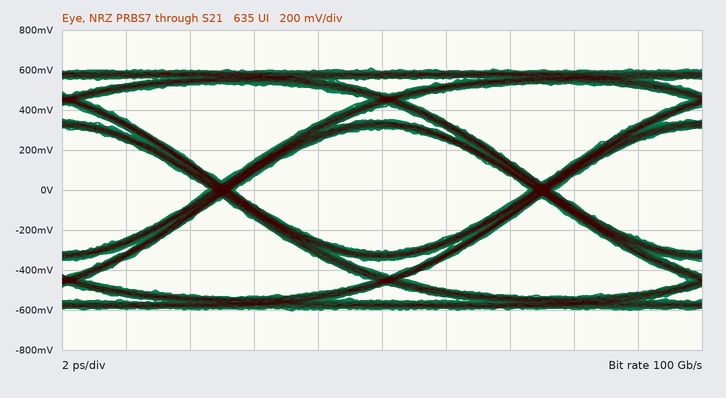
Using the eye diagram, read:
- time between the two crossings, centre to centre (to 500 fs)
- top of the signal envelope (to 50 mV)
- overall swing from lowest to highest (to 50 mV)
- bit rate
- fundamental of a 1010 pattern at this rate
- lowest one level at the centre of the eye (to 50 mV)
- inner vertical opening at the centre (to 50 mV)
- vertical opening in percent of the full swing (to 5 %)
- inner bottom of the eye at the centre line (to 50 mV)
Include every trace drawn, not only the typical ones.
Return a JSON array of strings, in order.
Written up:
["10.0 ps", "600 mV", "1.20 V", "100 Gb/s", "50 GHz", "300 mV", "600 mV", "50 %", "-300 mV"]
